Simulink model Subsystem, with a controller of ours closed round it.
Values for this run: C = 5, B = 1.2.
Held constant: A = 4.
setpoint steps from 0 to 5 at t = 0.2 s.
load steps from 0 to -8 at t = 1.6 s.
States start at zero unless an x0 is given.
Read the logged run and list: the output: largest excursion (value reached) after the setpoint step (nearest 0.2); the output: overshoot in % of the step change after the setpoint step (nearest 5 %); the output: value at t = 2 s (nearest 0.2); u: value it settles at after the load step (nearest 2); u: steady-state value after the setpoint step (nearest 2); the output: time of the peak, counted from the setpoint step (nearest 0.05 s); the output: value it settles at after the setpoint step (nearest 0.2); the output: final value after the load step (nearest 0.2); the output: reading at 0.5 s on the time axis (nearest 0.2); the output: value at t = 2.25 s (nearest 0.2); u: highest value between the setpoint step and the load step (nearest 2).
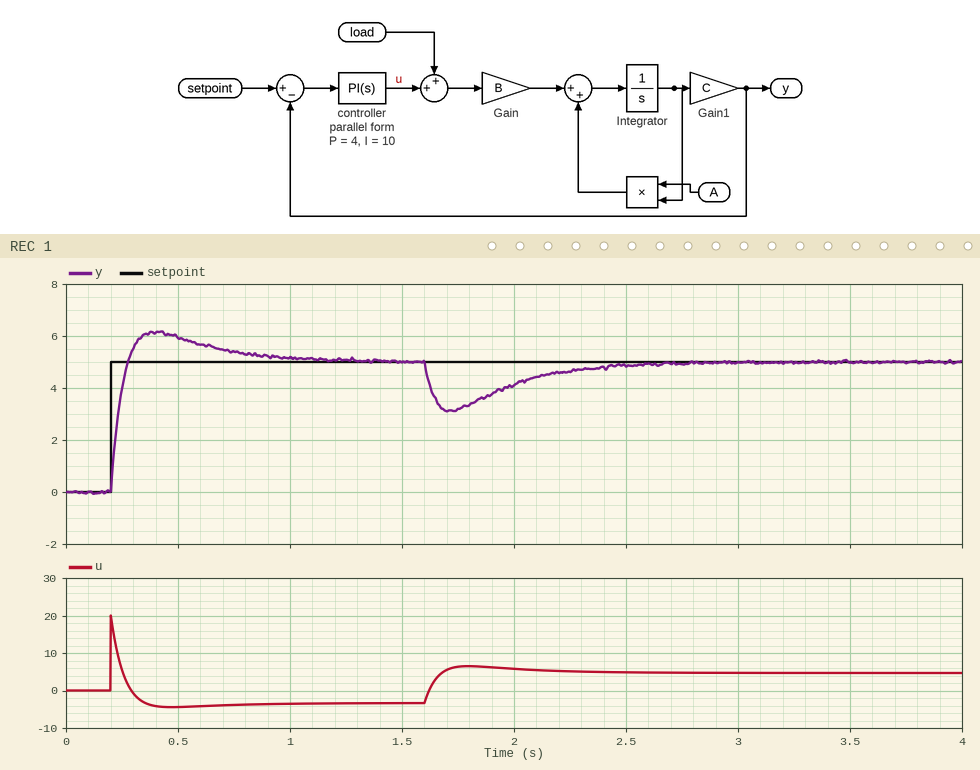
6.2
25 %
4.2
4
-4
0.20 s
5.0
5.0
6.0
4.6
20
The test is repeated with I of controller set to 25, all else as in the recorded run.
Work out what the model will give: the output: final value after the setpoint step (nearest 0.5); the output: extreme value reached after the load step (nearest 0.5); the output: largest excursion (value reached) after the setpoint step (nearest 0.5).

5.0
3.5
6.5
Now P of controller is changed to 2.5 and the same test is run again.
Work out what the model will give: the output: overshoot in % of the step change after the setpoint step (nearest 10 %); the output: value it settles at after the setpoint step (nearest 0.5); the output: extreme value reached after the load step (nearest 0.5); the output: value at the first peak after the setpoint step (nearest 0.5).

40 %
5.0
2.0
7.0
